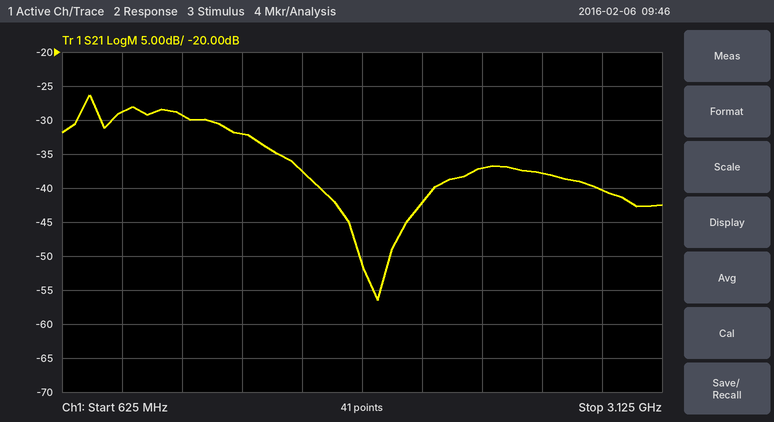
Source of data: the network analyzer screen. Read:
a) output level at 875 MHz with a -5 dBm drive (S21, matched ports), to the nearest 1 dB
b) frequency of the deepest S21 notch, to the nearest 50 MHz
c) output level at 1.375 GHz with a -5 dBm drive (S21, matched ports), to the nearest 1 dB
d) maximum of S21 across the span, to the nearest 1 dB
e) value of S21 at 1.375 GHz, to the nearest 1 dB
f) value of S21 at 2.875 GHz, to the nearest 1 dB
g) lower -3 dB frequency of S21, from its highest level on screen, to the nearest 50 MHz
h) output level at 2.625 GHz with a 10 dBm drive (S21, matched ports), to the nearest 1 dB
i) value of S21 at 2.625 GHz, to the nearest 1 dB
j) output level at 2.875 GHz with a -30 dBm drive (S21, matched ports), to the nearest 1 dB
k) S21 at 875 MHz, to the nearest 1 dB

-34 dBm
1.95 GHz
-37 dBm
-26 dB
-32 dB
-40 dB
700 MHz
-28 dBm
-38 dB
-70 dBm
-29 dB
